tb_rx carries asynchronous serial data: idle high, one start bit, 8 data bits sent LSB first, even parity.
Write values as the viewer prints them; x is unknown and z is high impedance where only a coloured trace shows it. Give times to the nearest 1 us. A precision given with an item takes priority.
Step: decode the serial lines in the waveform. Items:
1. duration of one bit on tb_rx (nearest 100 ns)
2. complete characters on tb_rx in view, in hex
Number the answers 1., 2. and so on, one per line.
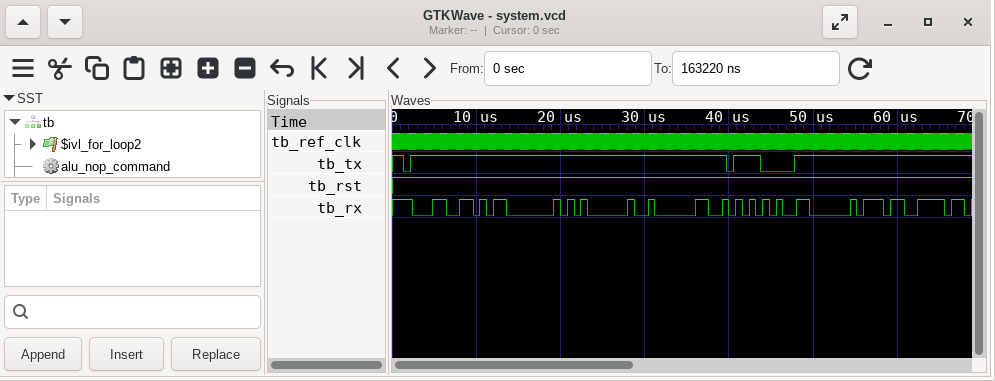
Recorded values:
1. 800 ns
2. CC, 03, 05, 02, AA, 06, 37
